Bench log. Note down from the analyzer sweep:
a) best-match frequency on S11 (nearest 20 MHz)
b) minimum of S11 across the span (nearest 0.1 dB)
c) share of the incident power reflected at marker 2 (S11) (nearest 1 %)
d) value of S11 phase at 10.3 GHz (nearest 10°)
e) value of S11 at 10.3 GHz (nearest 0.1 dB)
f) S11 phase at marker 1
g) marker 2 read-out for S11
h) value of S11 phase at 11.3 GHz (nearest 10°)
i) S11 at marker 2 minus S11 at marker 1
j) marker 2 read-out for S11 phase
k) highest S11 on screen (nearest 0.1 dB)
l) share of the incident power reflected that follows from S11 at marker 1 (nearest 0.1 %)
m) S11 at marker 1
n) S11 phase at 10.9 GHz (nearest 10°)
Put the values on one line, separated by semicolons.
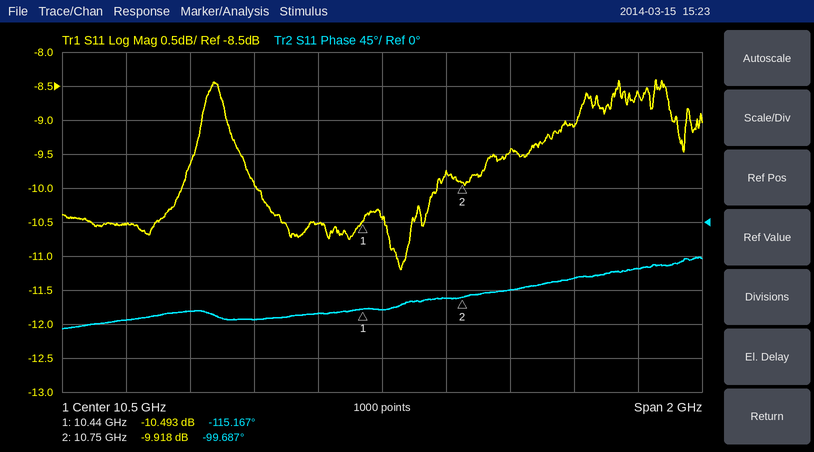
10.56 GHz; -11.2 dB; 10 %; -120°; -10.5 dB; -115.167°; -9.918 dB; -60°; 0.575 dB; -99.687°; -8.4 dB; 8.9 %; -10.493 dB; -90°
